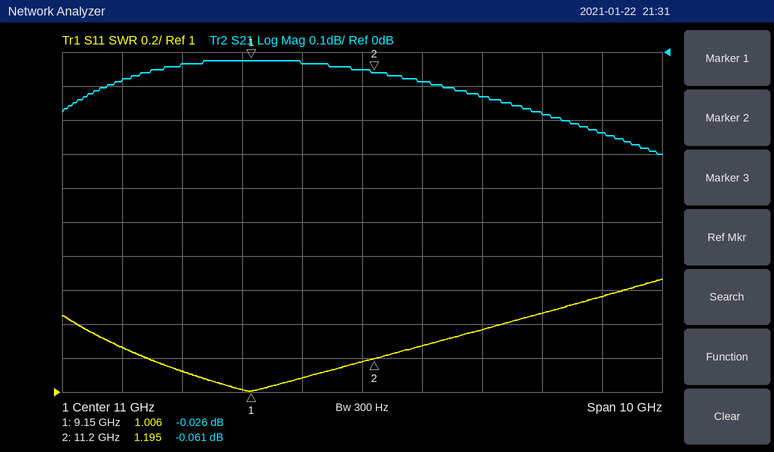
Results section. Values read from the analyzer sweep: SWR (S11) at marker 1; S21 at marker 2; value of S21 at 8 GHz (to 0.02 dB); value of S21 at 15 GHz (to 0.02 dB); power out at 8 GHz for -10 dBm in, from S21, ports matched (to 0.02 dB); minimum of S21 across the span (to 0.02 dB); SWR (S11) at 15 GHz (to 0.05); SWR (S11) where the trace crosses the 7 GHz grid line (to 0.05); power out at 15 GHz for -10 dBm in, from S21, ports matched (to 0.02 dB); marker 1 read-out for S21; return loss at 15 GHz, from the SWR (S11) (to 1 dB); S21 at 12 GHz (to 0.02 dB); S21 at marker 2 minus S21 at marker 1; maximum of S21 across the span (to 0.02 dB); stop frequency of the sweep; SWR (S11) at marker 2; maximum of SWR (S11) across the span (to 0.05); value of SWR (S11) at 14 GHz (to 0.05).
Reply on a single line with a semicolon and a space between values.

1.006; -0.061 dB; -0.04 dB; -0.24 dB; -10.04 dBm; -0.30 dB; 1.55; 1.25; -10.24 dBm; -0.026 dB; 13 dB; -0.08 dB; -0.035 dB; -0.02 dB; 16 GHz; 1.195; 1.65; 1.45
